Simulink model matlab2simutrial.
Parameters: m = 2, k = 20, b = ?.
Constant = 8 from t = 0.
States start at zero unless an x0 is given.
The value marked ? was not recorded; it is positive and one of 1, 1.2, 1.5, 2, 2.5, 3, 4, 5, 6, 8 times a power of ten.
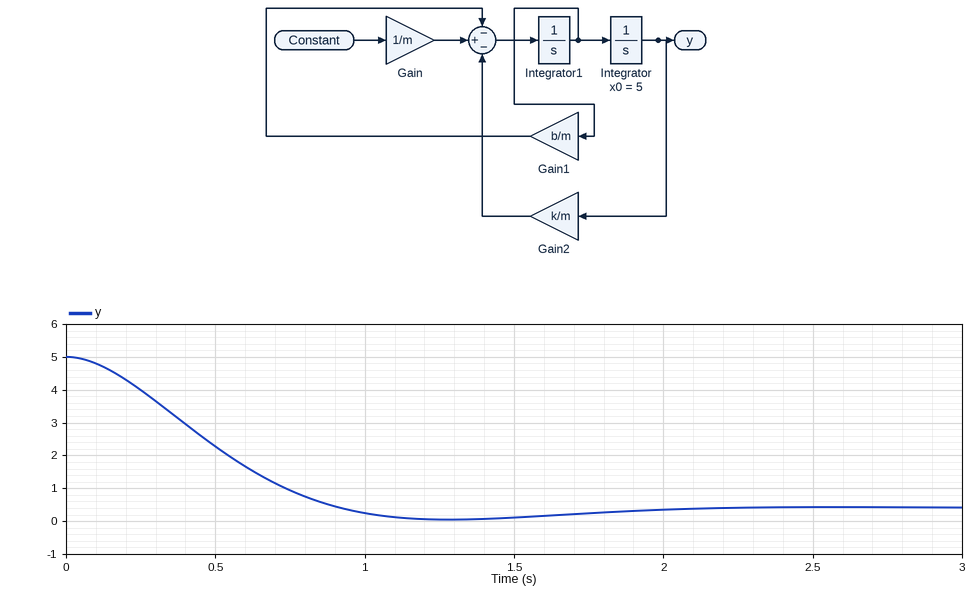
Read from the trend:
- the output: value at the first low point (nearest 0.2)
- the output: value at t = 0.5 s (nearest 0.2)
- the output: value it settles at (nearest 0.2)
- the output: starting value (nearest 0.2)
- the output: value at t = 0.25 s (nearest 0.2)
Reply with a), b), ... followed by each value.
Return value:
a) 0.0
b) 2.2
c) 0.4
d) 5.0
e) 4.0
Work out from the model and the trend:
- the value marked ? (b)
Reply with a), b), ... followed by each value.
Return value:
a) 8
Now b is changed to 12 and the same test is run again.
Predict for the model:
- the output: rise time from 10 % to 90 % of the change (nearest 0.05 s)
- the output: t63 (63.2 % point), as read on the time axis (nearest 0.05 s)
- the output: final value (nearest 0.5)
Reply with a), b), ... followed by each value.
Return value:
a) 1.00 s
b) 0.65 s
c) 0.5
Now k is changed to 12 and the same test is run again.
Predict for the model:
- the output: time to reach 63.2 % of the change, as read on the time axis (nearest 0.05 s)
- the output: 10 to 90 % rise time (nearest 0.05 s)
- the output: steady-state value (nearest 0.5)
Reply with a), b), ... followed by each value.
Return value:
a) 0.75 s
b) 1.05 s
c) 0.5
